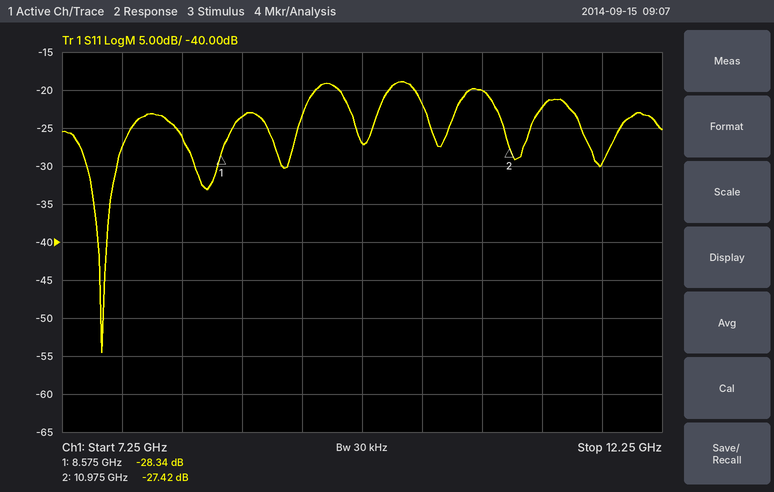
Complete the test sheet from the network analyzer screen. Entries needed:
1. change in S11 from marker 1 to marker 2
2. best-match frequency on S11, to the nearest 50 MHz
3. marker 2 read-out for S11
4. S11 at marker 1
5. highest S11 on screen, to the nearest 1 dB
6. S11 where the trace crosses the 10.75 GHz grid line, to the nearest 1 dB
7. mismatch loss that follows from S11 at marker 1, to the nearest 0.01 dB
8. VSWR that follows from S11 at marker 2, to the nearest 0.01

0.92 dB
7.60 GHz
-27.42 dB
-28.34 dB
-19 dB
-20 dB
0.01 dB
1.09
